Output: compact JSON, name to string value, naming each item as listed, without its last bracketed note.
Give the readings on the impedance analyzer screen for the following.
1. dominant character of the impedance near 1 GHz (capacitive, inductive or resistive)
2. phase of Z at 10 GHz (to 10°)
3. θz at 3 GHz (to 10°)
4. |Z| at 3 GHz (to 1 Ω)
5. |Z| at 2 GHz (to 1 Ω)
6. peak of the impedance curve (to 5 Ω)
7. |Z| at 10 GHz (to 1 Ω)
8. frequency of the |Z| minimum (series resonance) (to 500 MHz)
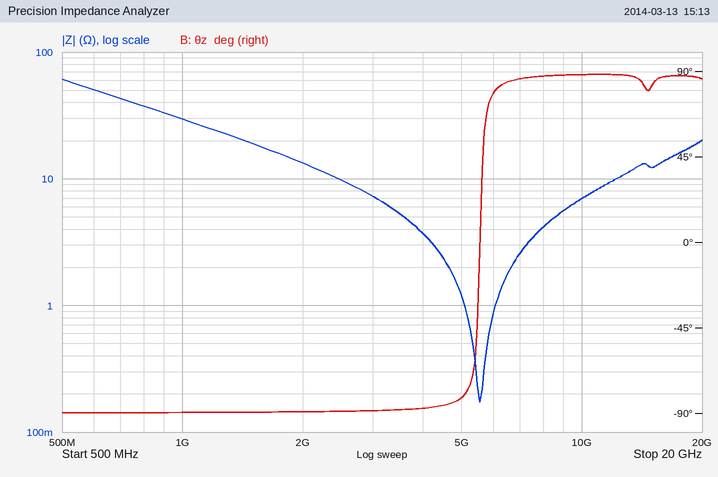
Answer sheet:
{"dominant character of the impedance near 1 GHz": "capacitive", "phase of Z at 10 GHz": "90°", "θz at 3 GHz": "-90°", "|Z| at 3 GHz": "7 Ω", "|Z| at 2 GHz": "13 Ω", "peak of the impedance curve": "60 Ω", "|Z| at 10 GHz": "7 Ω", "frequency of the |Z| minimum (series resonance)": "5.5 GHz"}
